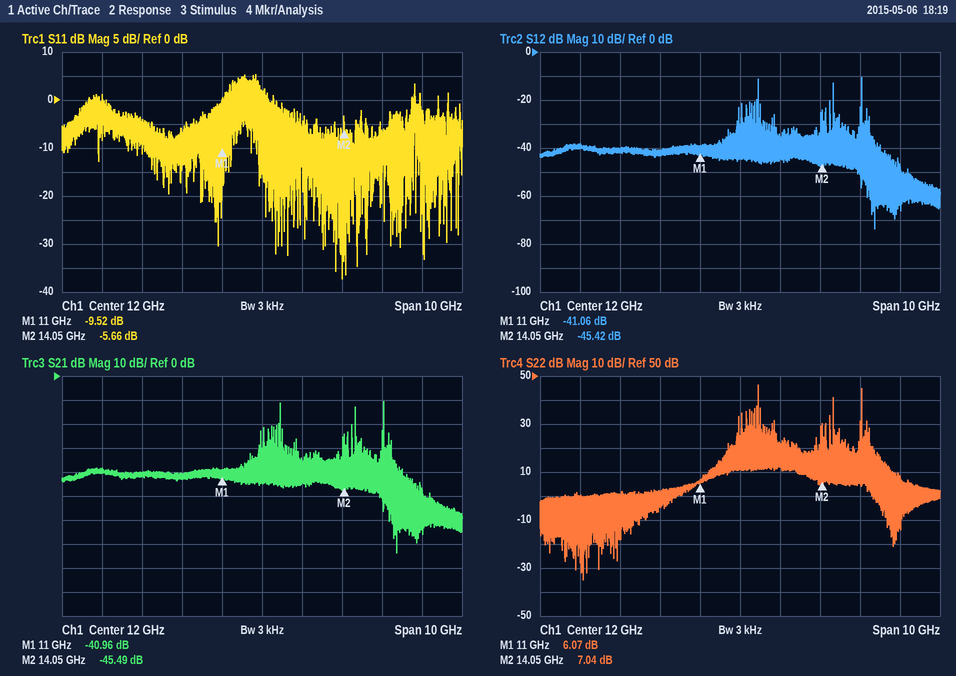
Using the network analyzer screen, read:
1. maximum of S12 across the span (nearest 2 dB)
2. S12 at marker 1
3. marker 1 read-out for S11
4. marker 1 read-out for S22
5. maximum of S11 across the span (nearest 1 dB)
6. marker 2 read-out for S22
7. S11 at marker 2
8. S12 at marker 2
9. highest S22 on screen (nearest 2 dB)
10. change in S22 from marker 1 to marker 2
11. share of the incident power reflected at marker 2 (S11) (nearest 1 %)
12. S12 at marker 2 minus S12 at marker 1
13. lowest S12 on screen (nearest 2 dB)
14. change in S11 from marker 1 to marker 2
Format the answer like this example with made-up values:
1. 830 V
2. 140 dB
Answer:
1. -10 dB
2. -41.06 dB
3. -9.52 dB
4. 6.07 dB
5. 5 dB
6. 7.04 dB
7. -5.66 dB
8. -45.42 dB
9. 46 dB
10. 0.97 dB
11. 27 %
12. -4.36 dB
13. -74 dB
14. 3.86 dB
